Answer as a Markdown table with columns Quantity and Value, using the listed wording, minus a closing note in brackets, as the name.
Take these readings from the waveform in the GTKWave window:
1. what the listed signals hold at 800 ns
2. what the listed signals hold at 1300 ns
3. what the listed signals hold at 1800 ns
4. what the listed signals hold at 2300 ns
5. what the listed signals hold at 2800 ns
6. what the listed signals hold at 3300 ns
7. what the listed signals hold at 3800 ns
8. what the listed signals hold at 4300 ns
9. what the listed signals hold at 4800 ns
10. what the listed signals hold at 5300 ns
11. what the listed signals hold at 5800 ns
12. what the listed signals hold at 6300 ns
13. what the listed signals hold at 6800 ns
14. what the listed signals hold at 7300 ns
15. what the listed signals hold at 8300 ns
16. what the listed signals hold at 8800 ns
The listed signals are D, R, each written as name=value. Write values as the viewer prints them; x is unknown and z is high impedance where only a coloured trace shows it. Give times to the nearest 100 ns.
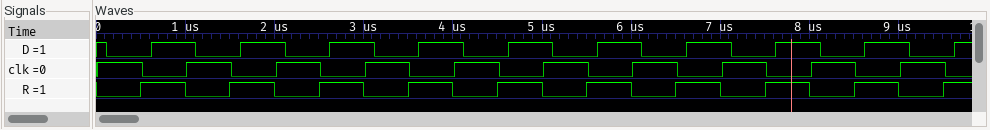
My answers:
| Quantity | Value |
|---|---|
| what the listed signals hold at 800 ns | D=1, R=1 |
| what the listed signals hold at 1300 ns | D=0, R=0 |
| what the listed signals hold at 1800 ns | D=1, R=1 |
| what the listed signals hold at 2300 ns | D=0, R=0 |
| what the listed signals hold at 2800 ns | D=1, R=1 |
| what the listed signals hold at 3300 ns | D=0, R=0 |
| what the listed signals hold at 3800 ns | D=1, R=1 |
| what the listed signals hold at 4300 ns | D=0, R=0 |
| what the listed signals hold at 4800 ns | D=1, R=1 |
| what the listed signals hold at 5300 ns | D=0, R=0 |
| what the listed signals hold at 5800 ns | D=1, R=1 |
| what the listed signals hold at 6300 ns | D=0, R=0 |
| what the listed signals hold at 6800 ns | D=1, R=1 |
| what the listed signals hold at 7300 ns | D=0, R=0 |
| what the listed signals hold at 8300 ns | D=0, R=0 |
| what the listed signals hold at 8800 ns | D=1, R=1 |
